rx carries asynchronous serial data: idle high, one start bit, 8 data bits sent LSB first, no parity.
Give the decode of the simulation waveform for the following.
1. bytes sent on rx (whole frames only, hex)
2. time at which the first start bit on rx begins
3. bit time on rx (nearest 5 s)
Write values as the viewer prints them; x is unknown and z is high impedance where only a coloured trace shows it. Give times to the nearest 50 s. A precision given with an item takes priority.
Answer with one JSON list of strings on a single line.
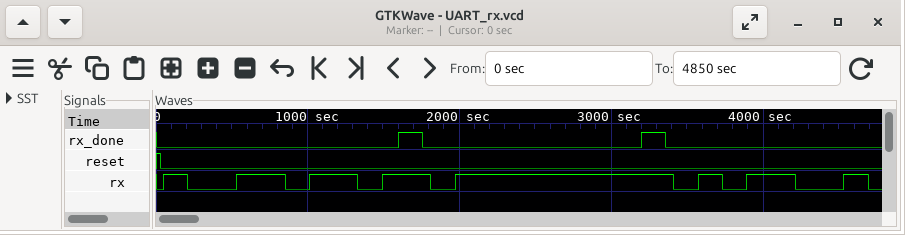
["B6, FF", "200 s", "160 s"]
